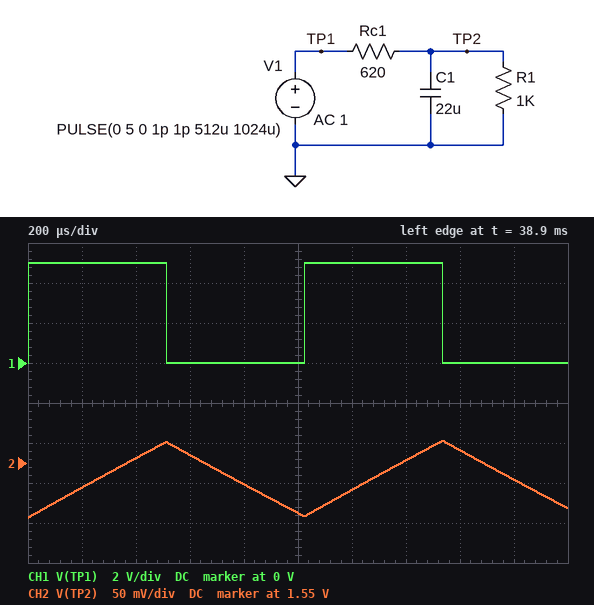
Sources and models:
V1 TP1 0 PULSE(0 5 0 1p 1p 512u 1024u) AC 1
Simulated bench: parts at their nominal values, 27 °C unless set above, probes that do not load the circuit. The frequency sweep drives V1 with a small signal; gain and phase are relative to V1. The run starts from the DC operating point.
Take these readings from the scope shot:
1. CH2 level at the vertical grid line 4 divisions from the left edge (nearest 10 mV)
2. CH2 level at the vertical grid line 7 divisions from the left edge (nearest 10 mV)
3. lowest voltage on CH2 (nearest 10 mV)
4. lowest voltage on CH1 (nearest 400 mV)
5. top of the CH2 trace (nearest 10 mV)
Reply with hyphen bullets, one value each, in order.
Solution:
- 1.52 V
- 1.55 V
- 1.48 V
- 0 V
- 1.58 V
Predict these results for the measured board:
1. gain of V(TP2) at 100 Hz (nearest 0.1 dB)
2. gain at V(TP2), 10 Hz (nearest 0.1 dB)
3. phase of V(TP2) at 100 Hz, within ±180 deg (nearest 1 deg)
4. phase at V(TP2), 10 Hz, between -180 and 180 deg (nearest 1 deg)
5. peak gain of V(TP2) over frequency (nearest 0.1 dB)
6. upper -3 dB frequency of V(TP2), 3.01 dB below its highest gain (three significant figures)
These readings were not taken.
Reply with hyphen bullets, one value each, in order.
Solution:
- -18.8 dB
- -5.3 dB
- -79 deg
- -28 deg
- -4.2 dB
- 18.9 Hz
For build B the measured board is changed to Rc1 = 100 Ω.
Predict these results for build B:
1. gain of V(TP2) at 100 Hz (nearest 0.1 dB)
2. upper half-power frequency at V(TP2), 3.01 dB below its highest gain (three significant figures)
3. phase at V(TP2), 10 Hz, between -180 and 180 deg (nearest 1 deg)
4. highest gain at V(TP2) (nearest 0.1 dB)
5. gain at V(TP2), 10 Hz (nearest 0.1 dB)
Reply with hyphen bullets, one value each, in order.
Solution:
- -4.9 dB
- 79.6 Hz
- -7 deg
- -0.8 dB
- -0.9 dB
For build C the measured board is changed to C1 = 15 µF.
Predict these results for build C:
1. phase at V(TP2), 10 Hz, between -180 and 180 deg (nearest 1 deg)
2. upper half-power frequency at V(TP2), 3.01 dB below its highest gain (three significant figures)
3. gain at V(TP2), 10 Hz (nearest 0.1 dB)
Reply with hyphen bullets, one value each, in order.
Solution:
- -20 deg
- 27.7 Hz
- -4.7 dB
